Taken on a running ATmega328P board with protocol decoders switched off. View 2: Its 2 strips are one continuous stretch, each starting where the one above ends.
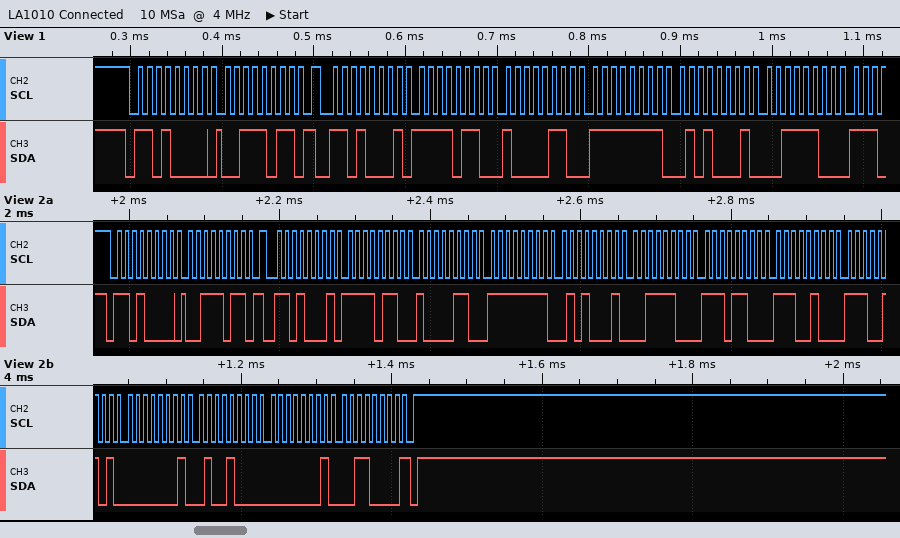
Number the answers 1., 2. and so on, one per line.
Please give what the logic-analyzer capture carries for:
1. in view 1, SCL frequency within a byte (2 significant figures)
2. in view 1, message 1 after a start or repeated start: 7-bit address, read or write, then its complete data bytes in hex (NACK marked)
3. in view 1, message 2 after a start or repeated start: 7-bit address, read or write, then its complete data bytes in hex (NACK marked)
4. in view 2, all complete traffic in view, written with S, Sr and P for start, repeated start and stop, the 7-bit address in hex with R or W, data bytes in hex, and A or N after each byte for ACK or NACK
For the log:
1. 100 kHz
2. 0x68 write: 3B
3. 0x68 read: F6 86 FF 51 3C
4. S 68W A 3B A Sr 68R A F6 A 86 A FF A 51 A 3C A EC A E4 A E5 A 01 A 48 A 01 A 30 N P
